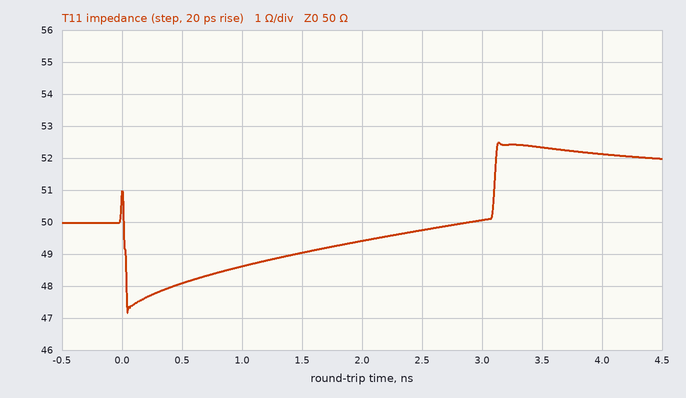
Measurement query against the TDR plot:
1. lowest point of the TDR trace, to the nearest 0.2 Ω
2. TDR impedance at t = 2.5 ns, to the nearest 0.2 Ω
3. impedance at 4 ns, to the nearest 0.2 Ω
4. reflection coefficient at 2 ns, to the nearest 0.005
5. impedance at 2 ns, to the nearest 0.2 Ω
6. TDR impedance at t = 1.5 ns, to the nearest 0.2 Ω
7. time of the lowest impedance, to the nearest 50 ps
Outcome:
47.2 Ω
49.8 Ω
52.2 Ω
-0.005
49.4 Ω
49.0 Ω
50 ps
